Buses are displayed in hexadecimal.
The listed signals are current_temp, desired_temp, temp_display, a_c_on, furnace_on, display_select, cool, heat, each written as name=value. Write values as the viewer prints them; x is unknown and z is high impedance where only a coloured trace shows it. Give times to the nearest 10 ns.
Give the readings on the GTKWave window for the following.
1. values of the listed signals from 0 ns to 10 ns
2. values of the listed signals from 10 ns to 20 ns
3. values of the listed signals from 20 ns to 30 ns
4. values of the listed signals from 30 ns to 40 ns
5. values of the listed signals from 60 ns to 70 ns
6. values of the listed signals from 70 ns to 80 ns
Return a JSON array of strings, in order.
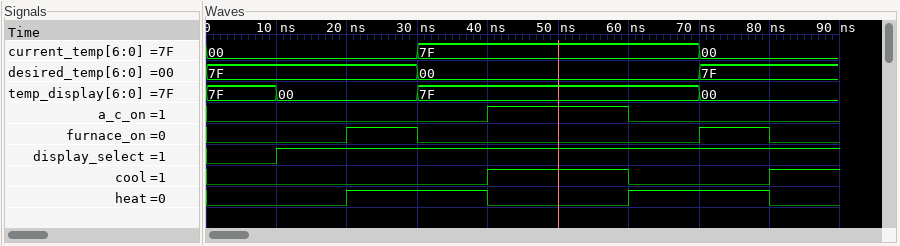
["current_temp=00, desired_temp=7F, temp_display=7F, a_c_on=0, furnace_on=0, display_select=0, cool=0, heat=0", "current_temp=00, desired_temp=7F, temp_display=00, a_c_on=0, furnace_on=0, display_select=1, cool=0, heat=0", "current_temp=00, desired_temp=7F, temp_display=00, a_c_on=0, furnace_on=1, display_select=1, cool=0, heat=1", "current_temp=7F, desired_temp=00, temp_display=7F, a_c_on=0, furnace_on=0, display_select=1, cool=0, heat=1", "current_temp=7F, desired_temp=00, temp_display=7F, a_c_on=0, furnace_on=0, display_select=1, cool=0, heat=1", "current_temp=00, desired_temp=7F, temp_display=00, a_c_on=0, furnace_on=1, display_select=1, cool=0, heat=1"]
